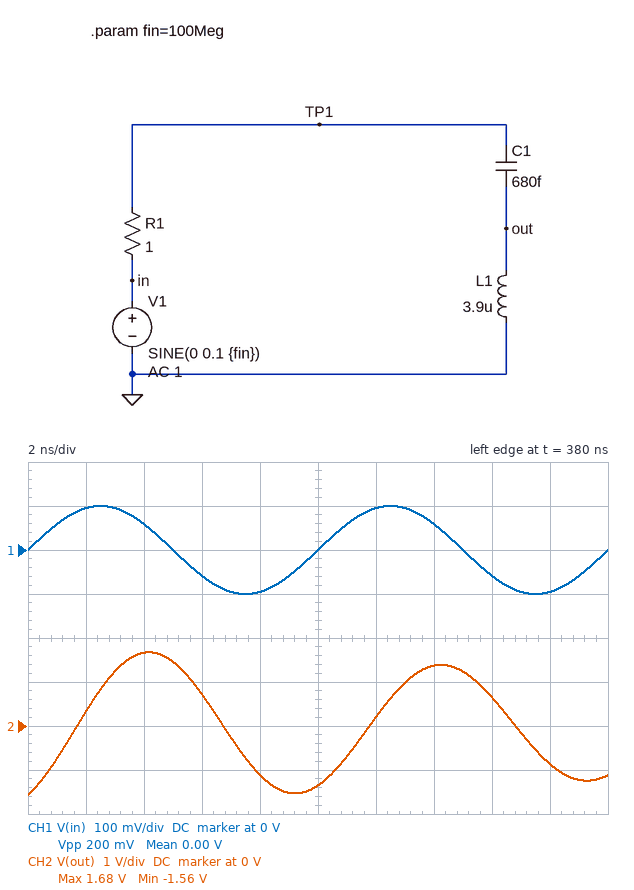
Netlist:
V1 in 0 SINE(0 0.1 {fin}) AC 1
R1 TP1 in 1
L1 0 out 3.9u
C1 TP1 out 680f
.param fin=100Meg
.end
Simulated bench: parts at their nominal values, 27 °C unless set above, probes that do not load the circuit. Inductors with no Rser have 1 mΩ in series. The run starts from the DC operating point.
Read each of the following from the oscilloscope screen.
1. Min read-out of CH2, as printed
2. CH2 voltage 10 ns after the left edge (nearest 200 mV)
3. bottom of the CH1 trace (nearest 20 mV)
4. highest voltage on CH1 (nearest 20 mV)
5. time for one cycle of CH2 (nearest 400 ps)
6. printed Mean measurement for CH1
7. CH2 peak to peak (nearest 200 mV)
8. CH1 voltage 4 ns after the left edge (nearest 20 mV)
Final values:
-1.56 V
-1.4 V
-100 mV
100 mV
10.0 ns
0.00 V
3.2 V
60 mV
